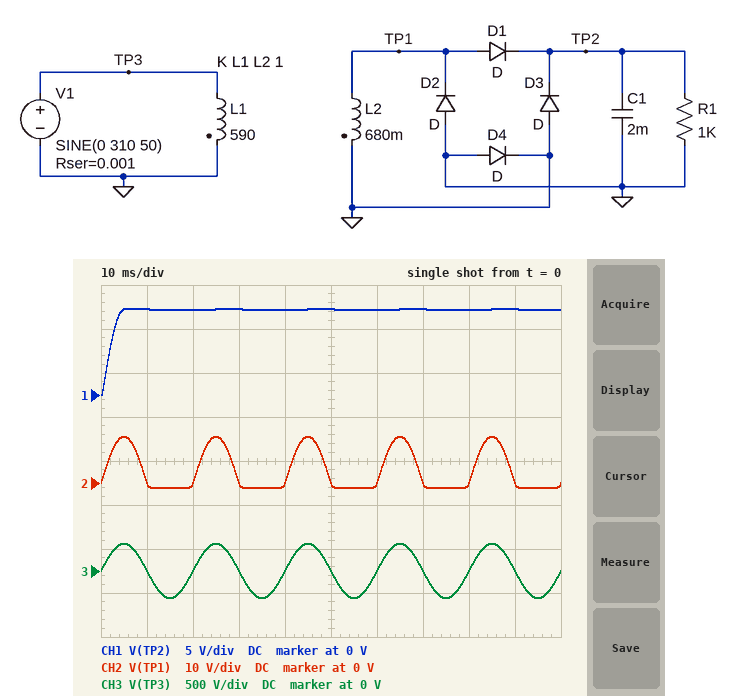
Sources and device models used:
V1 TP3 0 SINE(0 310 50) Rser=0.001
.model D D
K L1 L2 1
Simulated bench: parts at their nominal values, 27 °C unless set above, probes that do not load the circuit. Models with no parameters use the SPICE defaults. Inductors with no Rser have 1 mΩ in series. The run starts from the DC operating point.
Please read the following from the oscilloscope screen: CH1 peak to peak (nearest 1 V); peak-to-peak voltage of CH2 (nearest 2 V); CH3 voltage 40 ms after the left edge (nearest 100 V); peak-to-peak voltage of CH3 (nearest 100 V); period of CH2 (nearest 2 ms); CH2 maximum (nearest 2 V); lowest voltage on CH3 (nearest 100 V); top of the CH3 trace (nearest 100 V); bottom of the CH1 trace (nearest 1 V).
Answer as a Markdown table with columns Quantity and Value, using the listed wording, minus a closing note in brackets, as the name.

| Quantity | Value |
|---|---|
| CH1 peak to peak | 10 V |
| peak-to-peak voltage of CH2 | 12 V |
| CH3 voltage 40 ms after the left edge | 0 V |
| peak-to-peak voltage of CH3 | 600 V |
| period of CH2 | 20 ms |
| CH2 maximum | 10 V |
| lowest voltage on CH3 | -300 V |
| top of the CH3 trace | 300 V |
| bottom of the CH1 trace | 0 V |
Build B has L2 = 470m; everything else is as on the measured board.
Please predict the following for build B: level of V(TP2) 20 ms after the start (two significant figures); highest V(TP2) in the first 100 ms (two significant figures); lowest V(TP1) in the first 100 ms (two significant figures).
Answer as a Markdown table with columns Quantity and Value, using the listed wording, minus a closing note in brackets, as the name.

| Quantity | Value |
|---|---|
| level of V(TP2) 20 ms after the start | 7.9 V |
| highest V(TP2) in the first 100 ms | 8.0 V |
| lowest V(TP1) in the first 100 ms | -1.1 V |
